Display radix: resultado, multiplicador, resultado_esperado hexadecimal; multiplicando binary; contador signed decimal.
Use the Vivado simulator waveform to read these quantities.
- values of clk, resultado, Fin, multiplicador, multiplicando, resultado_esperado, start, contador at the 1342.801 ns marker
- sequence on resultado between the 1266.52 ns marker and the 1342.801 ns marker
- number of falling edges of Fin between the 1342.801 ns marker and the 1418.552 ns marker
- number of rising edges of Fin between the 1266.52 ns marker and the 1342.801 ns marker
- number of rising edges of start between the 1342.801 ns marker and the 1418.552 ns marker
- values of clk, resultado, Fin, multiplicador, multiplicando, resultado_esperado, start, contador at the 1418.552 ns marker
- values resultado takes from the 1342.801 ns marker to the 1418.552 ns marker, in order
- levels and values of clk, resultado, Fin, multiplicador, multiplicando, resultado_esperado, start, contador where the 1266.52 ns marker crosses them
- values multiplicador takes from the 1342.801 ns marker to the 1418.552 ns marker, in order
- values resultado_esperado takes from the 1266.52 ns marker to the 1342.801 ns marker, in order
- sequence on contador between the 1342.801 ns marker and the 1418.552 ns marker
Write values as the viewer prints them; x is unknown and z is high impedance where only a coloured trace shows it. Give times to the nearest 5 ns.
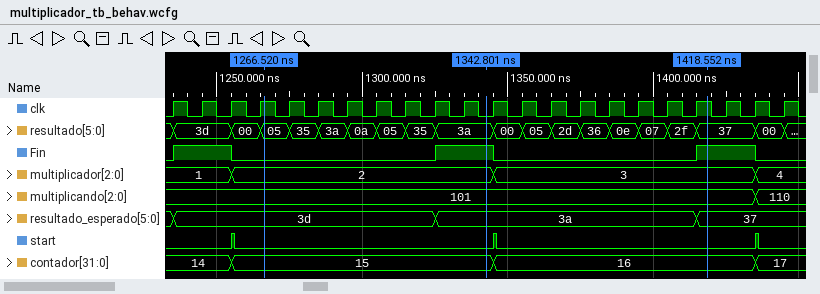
clk=0, resultado=3a, Fin=1, multiplicador=2, multiplicando=101, resultado_esperado=3a, start=0, contador=15
05, 35, 3a, 0a, 05, 35, 3a
1
1
1
clk=1, resultado=37, Fin=1, multiplicador=3, multiplicando=101, resultado_esperado=37, start=0, contador=16
3a, 00, 05, 2d, 36, 0e, 07, 2f, 37
clk=1, resultado=05, Fin=0, multiplicador=2, multiplicando=101, resultado_esperado=3d, start=0, contador=15
2, 3
3d, 3a
15, 16
